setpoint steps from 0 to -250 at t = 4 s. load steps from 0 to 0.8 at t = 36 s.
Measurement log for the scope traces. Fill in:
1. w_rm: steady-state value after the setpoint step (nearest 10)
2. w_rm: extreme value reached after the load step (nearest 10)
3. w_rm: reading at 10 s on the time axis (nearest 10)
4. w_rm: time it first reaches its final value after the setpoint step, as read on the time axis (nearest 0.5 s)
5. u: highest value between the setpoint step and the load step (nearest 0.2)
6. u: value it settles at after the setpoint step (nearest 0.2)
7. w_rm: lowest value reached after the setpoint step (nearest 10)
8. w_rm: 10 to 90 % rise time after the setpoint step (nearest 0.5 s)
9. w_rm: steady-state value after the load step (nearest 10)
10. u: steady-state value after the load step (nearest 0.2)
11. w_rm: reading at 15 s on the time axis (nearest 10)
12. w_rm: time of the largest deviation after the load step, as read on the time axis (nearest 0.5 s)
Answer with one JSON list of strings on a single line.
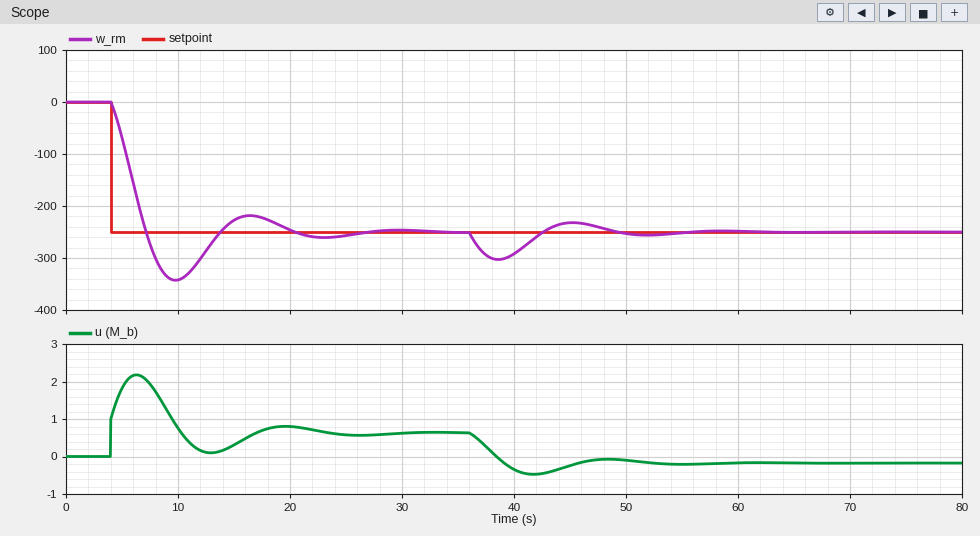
["-250", "-300", "-340", "7.0 s", "2.2", "0.6", "-340", "2.5 s", "-250", "-0.2", "-230", "38.5 s"]
